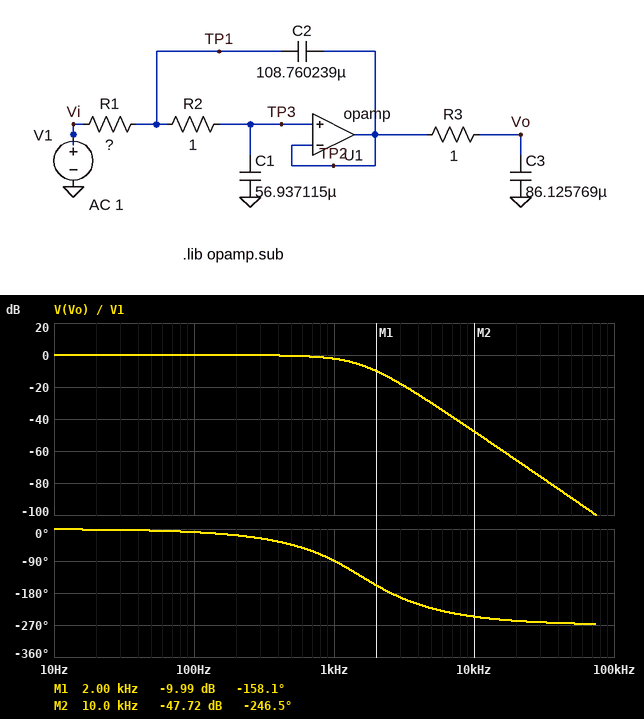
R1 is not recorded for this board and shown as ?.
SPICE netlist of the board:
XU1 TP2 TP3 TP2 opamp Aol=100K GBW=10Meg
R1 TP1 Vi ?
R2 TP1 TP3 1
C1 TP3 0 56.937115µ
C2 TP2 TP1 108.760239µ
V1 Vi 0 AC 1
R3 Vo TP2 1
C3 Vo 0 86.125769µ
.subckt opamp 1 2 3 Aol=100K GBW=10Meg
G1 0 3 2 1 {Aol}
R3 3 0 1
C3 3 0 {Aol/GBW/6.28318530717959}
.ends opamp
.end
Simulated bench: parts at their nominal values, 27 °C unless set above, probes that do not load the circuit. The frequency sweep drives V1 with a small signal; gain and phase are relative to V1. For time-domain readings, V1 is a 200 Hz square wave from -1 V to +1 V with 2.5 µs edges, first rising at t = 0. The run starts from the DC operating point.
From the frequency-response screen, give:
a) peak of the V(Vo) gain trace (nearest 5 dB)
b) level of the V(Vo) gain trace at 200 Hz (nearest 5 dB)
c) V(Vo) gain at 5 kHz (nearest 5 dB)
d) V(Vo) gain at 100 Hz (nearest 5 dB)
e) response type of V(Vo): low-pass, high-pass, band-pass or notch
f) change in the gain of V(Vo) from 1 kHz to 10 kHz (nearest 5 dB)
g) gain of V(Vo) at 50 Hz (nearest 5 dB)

0 dB
0 dB
-30 dB
0 dB
low-pass
-45 dB
0 dB
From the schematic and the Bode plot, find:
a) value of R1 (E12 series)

1.8 Ω
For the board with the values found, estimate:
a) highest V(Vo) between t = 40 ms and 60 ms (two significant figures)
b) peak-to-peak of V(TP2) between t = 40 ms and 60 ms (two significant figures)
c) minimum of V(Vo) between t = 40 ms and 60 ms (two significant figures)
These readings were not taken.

1.0 V
2.1 V
-1.0 V
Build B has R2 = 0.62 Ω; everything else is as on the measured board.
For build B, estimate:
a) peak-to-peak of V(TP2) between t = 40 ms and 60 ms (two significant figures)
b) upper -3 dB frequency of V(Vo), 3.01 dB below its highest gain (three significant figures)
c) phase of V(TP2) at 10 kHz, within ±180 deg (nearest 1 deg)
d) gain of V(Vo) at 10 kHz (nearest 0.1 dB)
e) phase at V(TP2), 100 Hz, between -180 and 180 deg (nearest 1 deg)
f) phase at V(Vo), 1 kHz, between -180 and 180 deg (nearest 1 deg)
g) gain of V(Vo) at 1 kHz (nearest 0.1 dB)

2.0 V
1.18 kHz
-162 deg
-43.7 dB
-5 deg
-78 deg
-2.2 dB
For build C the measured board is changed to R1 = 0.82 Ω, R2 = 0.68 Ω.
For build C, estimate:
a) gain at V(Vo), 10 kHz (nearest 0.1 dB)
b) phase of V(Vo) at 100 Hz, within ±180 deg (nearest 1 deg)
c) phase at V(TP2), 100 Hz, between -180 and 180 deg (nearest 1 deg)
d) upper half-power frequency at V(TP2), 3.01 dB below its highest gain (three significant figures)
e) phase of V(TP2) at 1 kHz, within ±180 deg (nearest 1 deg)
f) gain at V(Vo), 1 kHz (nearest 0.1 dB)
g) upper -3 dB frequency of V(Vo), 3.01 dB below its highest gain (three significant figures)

-37.6 dB
-6 deg
-3 deg
2.63 kHz
-32 deg
-1.3 dB
1.58 kHz
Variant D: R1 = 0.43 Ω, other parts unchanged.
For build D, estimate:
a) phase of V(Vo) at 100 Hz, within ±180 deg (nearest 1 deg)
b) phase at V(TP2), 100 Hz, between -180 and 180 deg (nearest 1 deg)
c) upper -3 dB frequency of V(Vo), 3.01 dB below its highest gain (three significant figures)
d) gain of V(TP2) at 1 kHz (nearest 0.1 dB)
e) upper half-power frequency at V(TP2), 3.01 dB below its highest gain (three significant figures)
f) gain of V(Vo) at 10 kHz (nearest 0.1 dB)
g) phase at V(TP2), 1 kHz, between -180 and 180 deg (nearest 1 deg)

-6 deg
-3 deg
1.54 kHz
-0.3 dB
2.73 kHz
-35.5 dB
-30 deg
